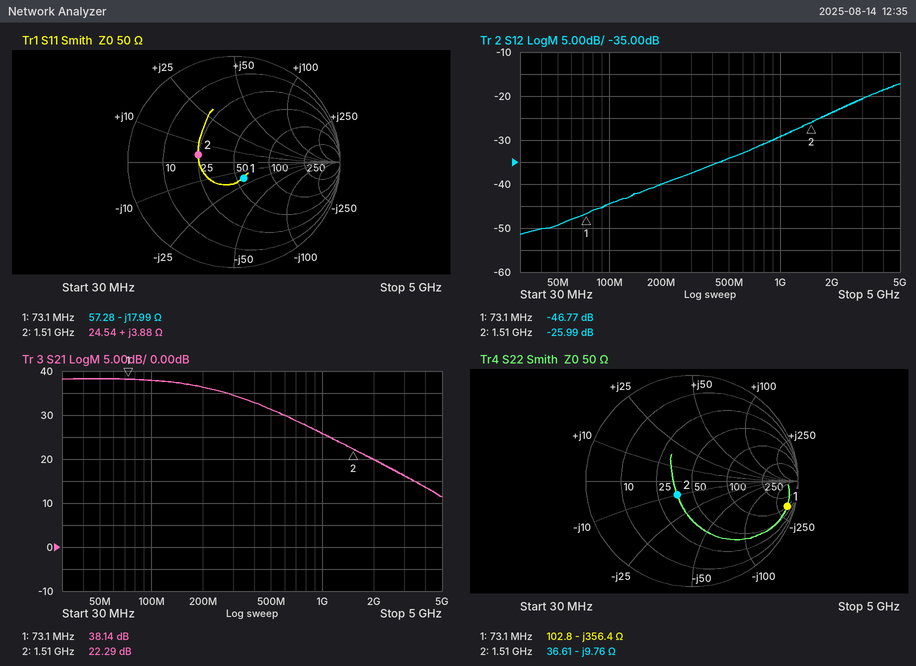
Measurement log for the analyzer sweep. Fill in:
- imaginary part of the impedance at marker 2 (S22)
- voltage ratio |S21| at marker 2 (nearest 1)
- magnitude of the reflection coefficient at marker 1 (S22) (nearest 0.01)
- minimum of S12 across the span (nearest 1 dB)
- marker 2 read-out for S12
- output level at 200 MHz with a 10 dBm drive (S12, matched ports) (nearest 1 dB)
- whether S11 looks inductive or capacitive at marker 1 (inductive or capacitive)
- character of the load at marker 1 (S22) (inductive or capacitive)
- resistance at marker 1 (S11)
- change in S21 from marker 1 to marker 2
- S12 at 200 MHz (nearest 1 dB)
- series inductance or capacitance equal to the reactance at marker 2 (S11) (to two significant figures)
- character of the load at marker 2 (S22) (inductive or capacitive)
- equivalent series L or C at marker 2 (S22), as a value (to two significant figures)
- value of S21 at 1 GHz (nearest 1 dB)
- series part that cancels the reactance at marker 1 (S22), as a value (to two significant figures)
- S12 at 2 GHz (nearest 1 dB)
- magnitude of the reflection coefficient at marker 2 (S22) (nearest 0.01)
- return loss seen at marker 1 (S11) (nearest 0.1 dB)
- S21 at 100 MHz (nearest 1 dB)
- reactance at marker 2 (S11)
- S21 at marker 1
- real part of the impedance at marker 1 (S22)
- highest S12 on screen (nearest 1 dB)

-9.76 Ω
13
0.93
-51 dB
-25.99 dB
-30 dBm
capacitive
capacitive
57.28 Ω
-15.85 dB
-40 dB
410 pH
capacitive
11 pF
26 dB
780 nH
-24 dB
0.19
15.0 dB
38 dB
+3.88 Ω
38.14 dB
102.8 Ω
-17 dB
